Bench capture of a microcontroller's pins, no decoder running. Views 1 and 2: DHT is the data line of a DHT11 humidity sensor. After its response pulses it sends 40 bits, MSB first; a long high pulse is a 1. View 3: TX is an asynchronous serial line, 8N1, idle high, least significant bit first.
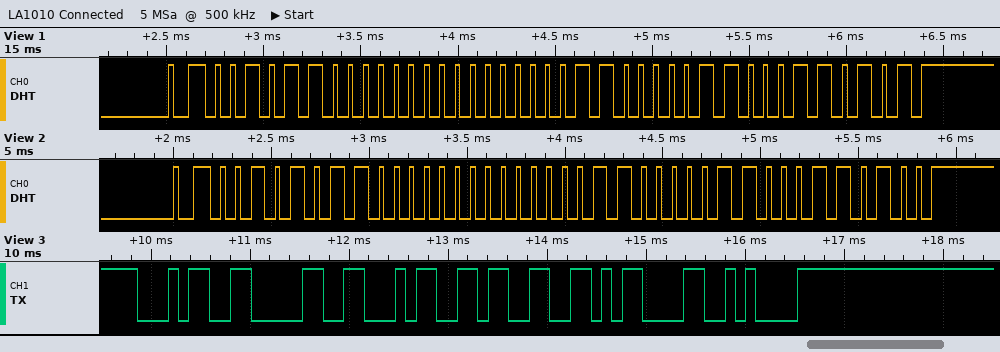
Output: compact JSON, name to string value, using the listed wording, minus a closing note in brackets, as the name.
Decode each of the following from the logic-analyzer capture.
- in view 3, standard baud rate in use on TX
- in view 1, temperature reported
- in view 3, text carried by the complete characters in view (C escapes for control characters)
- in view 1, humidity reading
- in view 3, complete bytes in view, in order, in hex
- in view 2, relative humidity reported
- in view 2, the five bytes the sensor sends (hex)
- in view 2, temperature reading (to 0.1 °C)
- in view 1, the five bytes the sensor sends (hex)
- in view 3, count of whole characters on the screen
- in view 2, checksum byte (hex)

{"in view 3, standard baud rate in use on TX": "9600 baud", "in view 1, temperature reported": "3.6 °C", "in view 3, text carried by the complete characters in view": "\"4043\\r\\n\"", "in view 1, humidity reading": "44 %", "in view 3, complete bytes in view, in order, in hex": "0x34 0x30 0x34 0x33 0x0D 0x0A", "in view 2, relative humidity reported": "43 %", "in view 2, the five bytes the sensor sends": "2B 00 03 06 34", "in view 2, temperature reading": "3.6 °C", "in view 1, the five bytes the sensor sends": "2C 00 03 06 35", "in view 3, count of whole characters on the screen": "6", "in view 2, checksum byte": "0x34"}
